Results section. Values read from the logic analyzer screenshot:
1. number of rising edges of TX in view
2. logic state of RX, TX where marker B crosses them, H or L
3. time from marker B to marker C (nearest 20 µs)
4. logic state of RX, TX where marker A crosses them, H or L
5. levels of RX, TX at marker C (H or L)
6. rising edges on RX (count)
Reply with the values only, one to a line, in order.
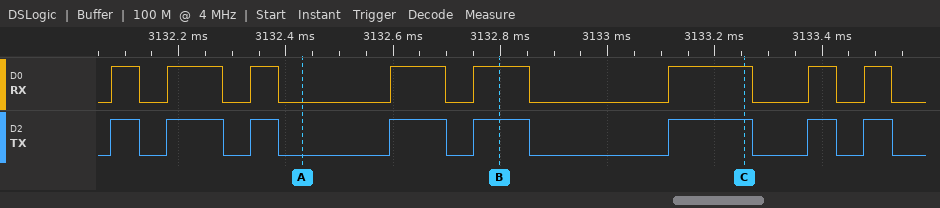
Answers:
8
RX=H, TX=H
460 µs
RX=L, TX=L
RX=H, TX=H
8
